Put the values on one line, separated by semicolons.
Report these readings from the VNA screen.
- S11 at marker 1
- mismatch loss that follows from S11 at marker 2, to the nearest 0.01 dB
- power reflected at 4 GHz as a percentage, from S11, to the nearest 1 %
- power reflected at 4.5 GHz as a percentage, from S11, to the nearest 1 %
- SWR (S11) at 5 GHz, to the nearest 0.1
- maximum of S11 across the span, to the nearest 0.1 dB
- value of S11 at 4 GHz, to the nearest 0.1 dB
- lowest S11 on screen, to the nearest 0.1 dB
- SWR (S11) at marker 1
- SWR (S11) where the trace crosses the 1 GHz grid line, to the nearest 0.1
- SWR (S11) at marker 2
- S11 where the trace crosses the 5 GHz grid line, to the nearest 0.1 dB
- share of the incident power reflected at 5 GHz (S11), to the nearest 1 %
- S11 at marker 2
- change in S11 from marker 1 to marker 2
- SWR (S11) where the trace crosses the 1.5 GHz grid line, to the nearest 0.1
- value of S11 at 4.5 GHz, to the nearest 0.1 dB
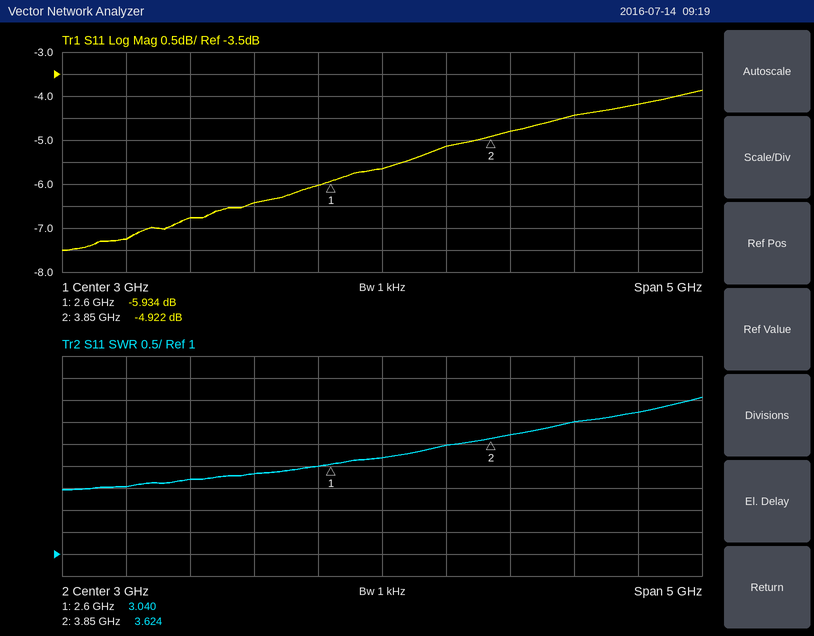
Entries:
-5.934 dB; 1.69 dB; 33 %; 36 %; 4.2; -3.9 dB; -4.8 dB; -7.5 dB; 3.040; 2.5; 3.624; -4.2 dB; 38 %; -4.922 dB; 1.012 dB; 2.7; -4.4 dB
